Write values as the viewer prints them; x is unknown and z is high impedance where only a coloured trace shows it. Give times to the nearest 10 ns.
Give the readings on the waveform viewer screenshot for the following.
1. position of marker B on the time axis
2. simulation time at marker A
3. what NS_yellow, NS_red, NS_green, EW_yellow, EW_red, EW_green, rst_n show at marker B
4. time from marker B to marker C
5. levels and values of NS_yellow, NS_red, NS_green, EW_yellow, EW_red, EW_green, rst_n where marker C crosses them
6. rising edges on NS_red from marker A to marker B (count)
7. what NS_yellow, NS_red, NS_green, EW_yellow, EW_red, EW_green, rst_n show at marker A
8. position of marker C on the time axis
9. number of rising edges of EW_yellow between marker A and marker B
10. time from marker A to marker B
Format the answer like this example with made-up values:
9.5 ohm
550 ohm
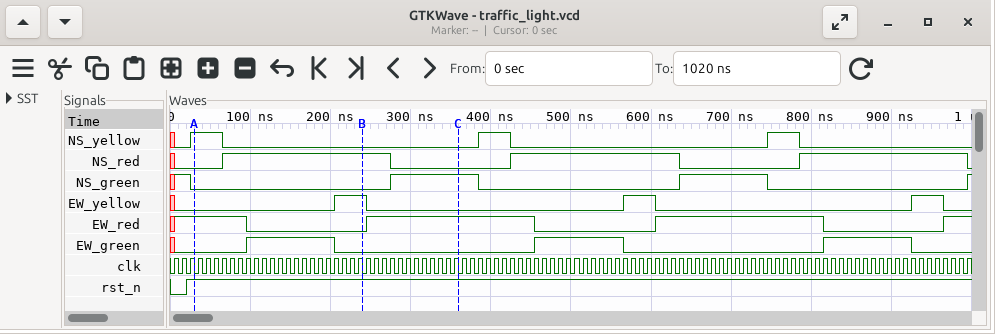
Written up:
240 ns
30 ns
NS_yellow=0, NS_red=1, NS_green=0, EW_yellow=1, EW_red=0, EW_green=0, rst_n=1
120 ns
NS_yellow=0, NS_red=0, NS_green=1, EW_yellow=0, EW_red=1, EW_green=0, rst_n=1
1
NS_yellow=1, NS_red=0, NS_green=0, EW_yellow=0, EW_red=1, EW_green=0, rst_n=1
360 ns
1
210 ns
